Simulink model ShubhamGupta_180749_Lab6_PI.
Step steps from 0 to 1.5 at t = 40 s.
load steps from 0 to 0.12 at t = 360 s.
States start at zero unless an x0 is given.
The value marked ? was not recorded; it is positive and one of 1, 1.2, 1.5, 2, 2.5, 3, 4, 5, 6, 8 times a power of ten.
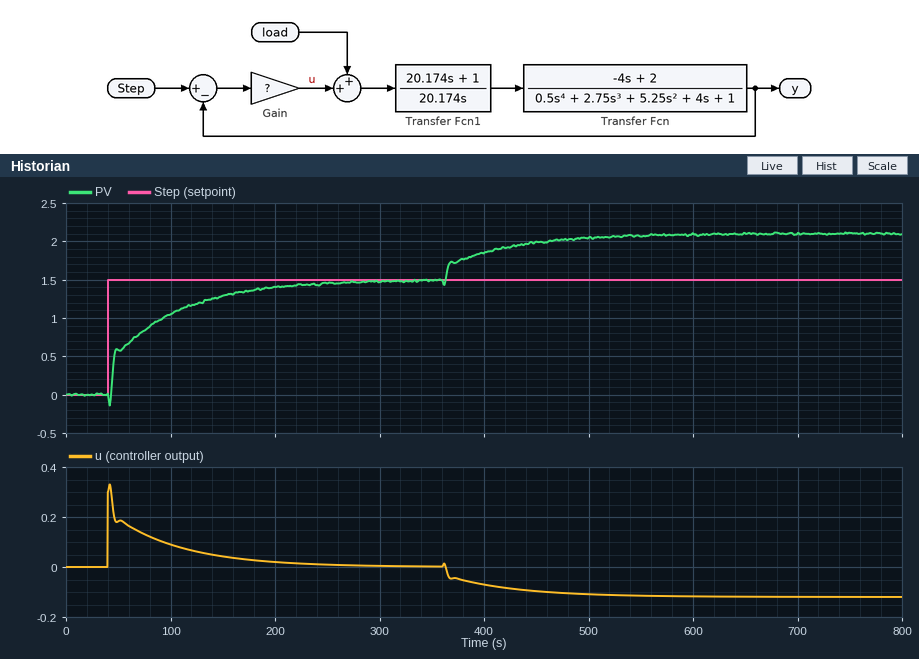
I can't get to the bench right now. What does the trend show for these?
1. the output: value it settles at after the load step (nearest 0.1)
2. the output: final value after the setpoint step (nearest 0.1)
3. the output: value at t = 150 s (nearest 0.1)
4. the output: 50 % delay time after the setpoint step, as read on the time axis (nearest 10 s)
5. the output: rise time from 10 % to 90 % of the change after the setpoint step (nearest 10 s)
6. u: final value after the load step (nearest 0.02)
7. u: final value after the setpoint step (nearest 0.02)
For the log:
2.1
1.5
1.3
70 s
130 s
-0.12
0.00
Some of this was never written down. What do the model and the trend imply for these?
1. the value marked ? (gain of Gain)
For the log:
0.2
